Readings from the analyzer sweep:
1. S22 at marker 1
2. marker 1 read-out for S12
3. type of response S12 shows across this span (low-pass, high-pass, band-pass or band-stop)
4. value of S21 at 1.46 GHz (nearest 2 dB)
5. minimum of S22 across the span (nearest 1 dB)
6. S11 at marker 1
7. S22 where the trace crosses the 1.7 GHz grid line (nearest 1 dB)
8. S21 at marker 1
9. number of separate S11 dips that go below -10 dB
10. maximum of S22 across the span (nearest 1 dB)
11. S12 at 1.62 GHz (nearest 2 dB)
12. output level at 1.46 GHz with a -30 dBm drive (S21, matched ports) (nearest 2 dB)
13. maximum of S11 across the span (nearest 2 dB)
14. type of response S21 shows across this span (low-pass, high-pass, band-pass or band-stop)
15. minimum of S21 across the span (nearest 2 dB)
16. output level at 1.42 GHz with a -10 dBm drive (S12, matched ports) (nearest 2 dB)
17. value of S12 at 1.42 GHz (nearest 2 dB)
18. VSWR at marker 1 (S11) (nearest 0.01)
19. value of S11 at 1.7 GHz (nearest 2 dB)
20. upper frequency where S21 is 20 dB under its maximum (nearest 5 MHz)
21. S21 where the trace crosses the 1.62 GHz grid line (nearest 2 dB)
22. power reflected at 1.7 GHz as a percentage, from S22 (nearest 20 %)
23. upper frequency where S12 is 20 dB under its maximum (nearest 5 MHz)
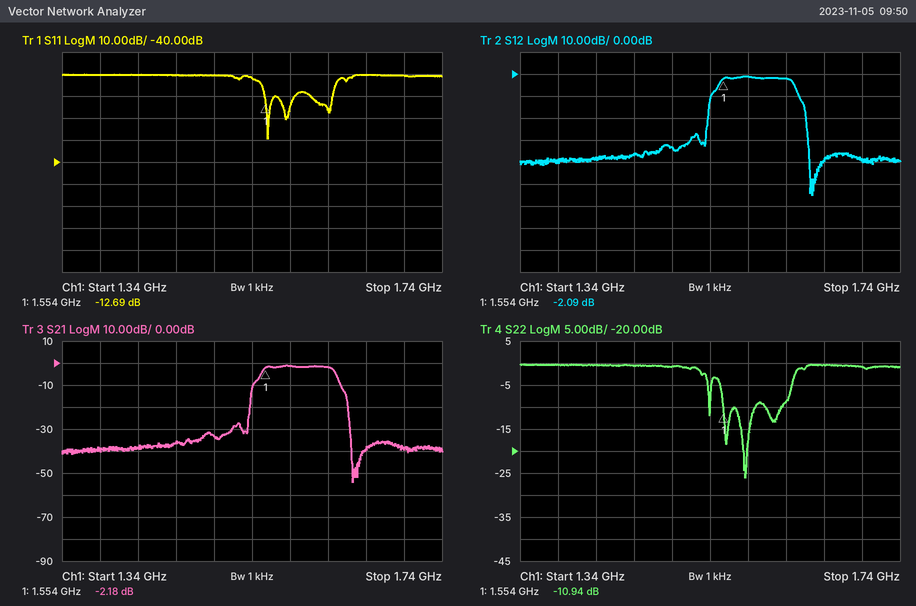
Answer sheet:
-10.94 dB
-2.09 dB
band-pass
-36 dB
-26 dB
-12.69 dB
-1 dB
-2.18 dB
3
0 dB
-2 dB
-66 dBm
0 dB
band-pass
-54 dB
-48 dBm
-38 dB
1.60
0 dB
1.640 GHz
-2 dB
80 %
1.640 GHz
